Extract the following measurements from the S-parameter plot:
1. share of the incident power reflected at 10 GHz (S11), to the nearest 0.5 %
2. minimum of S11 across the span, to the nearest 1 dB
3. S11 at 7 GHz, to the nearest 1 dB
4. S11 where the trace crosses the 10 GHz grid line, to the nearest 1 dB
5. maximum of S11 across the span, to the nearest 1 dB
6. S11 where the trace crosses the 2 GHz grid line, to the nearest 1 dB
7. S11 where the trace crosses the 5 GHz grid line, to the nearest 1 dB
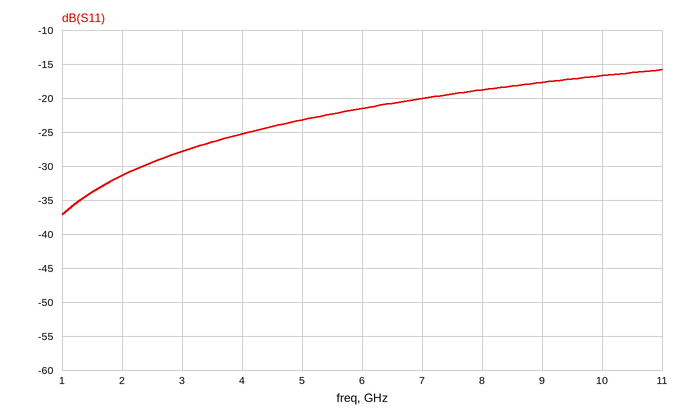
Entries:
2.0 %
-37 dB
-20 dB
-17 dB
-16 dB
-31 dB
-23 dB
